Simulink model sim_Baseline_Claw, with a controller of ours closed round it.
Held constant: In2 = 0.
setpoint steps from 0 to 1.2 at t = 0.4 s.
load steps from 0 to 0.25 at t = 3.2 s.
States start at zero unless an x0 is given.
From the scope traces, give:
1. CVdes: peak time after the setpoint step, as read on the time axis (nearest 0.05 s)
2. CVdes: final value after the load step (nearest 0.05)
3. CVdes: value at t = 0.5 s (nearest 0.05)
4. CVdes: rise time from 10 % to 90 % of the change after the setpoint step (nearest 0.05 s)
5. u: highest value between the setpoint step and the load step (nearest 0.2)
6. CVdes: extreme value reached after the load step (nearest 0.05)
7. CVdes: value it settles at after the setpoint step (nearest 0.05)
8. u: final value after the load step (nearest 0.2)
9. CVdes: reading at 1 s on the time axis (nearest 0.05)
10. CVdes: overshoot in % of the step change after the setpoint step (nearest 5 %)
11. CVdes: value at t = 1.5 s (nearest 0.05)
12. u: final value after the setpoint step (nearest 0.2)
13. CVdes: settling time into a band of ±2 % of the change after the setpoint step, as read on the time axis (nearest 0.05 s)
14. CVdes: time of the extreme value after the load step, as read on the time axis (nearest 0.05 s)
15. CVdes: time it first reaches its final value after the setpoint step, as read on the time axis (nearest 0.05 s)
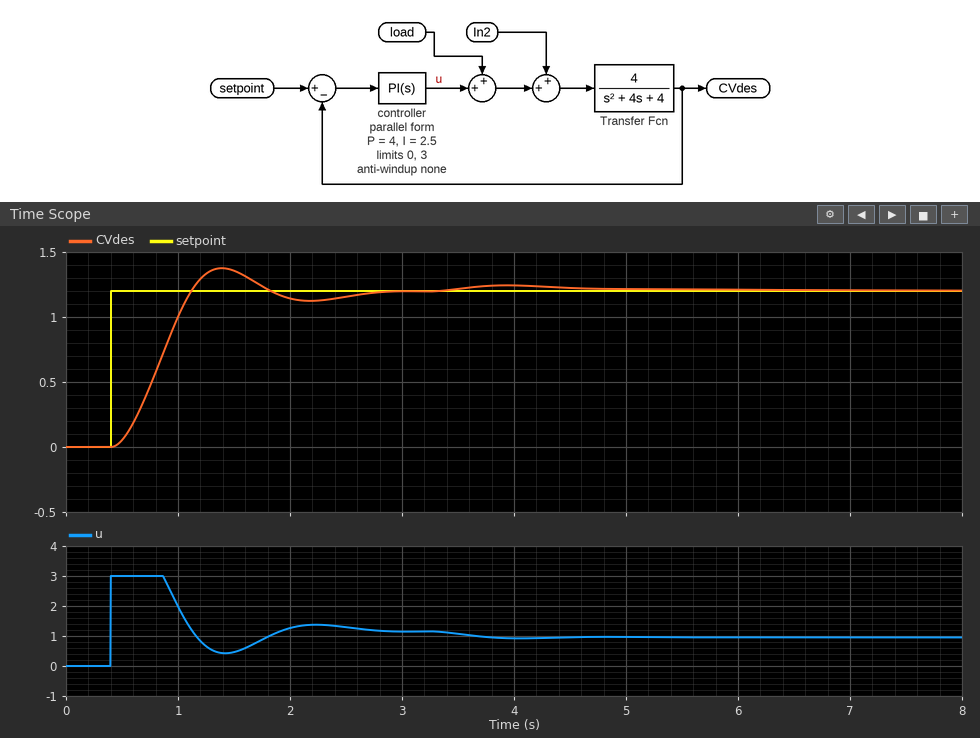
1.40 s
1.20
0.05
0.50 s
3.0
1.25
1.20
1.0
1.00
15 %
1.35
1.2
2.65 s
3.95 s
1.10 s
